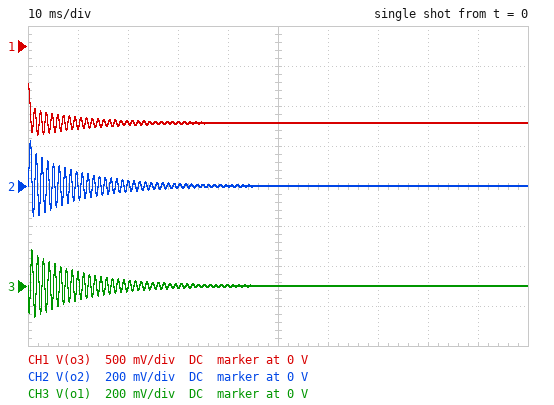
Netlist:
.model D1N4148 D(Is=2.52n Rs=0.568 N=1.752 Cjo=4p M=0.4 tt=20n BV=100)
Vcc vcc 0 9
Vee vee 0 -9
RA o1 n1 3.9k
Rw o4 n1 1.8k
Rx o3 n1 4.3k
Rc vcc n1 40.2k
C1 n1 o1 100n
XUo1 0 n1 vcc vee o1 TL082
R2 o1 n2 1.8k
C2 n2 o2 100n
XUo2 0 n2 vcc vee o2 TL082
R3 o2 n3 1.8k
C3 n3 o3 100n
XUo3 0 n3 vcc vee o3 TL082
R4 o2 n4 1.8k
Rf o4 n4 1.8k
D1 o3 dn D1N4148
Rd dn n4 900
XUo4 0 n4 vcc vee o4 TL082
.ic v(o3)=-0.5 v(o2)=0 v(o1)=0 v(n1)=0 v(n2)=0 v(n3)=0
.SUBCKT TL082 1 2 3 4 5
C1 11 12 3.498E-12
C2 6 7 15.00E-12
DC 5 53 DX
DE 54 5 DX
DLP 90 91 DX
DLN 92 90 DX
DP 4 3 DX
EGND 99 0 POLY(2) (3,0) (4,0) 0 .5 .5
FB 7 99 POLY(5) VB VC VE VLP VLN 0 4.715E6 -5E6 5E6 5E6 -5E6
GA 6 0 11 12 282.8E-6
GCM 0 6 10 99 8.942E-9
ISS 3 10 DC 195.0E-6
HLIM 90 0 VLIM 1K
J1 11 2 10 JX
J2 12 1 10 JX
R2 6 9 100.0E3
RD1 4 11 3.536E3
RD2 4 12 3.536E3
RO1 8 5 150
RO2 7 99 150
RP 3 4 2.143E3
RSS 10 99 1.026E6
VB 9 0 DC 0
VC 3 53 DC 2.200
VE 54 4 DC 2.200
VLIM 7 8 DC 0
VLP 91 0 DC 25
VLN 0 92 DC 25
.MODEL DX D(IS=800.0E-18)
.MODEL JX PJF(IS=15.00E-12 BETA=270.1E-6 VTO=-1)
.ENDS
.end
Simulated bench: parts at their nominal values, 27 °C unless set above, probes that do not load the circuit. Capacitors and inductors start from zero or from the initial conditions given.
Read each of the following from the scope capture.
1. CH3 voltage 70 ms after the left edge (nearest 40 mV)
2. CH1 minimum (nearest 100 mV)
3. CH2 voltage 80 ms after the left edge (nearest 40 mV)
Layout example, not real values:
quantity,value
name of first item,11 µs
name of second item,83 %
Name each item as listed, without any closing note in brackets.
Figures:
quantity,value
CH3 voltage 70 ms after the left edge,0 V
CH1 minimum,-1.1 V
CH2 voltage 80 ms after the left edge,0 V
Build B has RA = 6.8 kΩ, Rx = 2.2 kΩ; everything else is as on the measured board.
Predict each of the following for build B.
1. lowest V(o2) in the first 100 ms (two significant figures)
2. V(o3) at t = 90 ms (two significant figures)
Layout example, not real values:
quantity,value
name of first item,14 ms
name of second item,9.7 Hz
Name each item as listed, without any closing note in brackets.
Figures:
quantity,value
lowest V(o2) in the first 100 ms,-7.5 V
V(o3) at t = 90 ms,7.5 V
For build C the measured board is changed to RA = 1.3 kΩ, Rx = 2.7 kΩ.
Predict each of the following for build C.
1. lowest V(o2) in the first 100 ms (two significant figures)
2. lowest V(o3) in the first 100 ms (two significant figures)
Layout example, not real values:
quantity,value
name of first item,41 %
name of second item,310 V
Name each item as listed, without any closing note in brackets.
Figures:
quantity,value
lowest V(o2) in the first 100 ms,-24 mV
lowest V(o3) in the first 100 ms,-640 mV
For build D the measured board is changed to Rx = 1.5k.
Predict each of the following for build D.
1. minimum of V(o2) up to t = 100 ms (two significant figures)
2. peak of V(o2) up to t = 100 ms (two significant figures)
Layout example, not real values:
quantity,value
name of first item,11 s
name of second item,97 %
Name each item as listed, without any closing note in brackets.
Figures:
quantity,value
minimum of V(o2) up to t = 100 ms,-7.5 V
peak of V(o2) up to t = 100 ms,6.5 V
